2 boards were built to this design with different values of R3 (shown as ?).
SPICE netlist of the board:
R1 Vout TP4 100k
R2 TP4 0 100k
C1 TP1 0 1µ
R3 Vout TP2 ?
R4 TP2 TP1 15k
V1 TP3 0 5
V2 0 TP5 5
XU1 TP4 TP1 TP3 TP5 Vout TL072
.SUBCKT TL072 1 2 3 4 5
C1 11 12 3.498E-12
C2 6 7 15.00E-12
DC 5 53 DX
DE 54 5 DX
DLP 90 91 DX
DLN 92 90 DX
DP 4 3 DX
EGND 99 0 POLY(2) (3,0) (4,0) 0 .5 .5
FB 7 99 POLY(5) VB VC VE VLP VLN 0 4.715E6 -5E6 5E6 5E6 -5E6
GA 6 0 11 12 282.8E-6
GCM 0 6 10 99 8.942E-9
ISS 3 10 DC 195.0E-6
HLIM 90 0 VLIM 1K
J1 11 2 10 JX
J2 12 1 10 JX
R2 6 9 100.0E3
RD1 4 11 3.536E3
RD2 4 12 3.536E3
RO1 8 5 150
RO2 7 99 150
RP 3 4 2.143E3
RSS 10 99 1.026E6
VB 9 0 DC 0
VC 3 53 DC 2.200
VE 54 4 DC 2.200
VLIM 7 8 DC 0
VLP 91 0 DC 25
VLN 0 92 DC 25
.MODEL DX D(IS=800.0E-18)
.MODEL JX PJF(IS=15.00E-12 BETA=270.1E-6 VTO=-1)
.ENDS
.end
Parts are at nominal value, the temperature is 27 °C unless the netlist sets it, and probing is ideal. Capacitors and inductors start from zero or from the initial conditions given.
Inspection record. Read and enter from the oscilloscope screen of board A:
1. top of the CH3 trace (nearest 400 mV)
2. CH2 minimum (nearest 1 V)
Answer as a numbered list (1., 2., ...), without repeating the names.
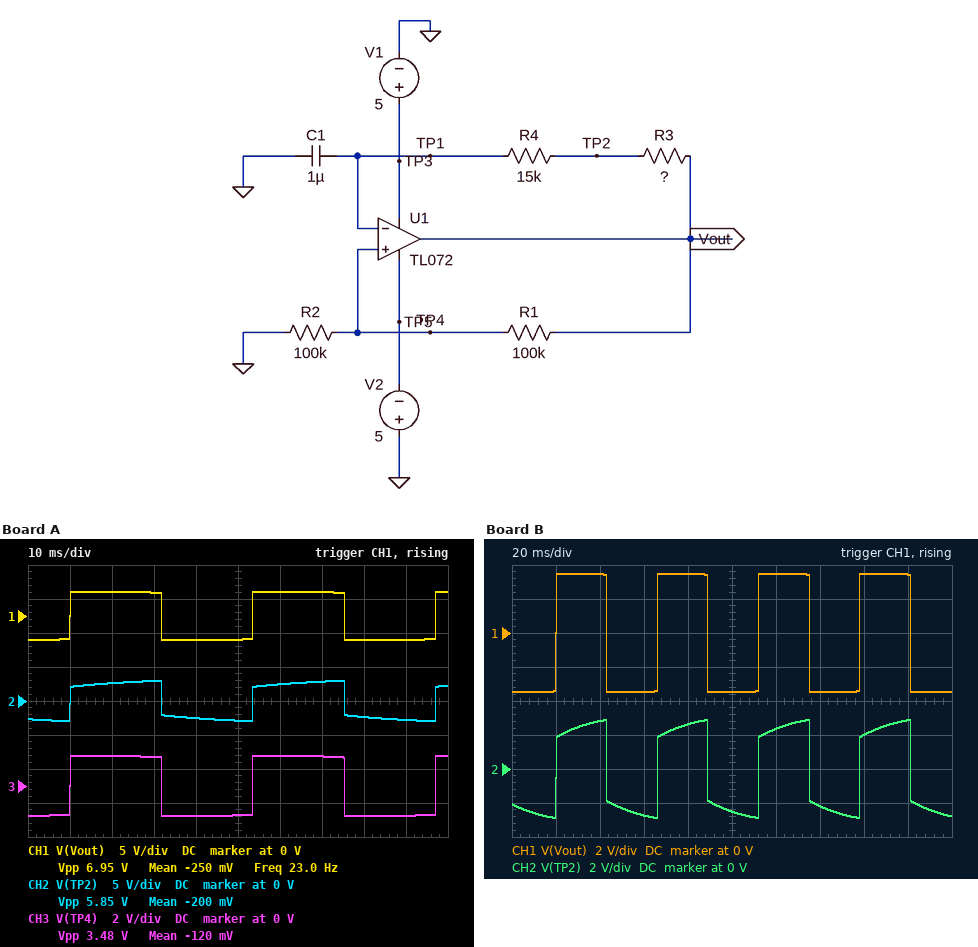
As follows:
1. 1.6 V
2. -3 V
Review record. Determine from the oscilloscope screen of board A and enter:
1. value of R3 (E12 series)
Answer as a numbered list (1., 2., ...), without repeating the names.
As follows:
1. 5.6 kΩ
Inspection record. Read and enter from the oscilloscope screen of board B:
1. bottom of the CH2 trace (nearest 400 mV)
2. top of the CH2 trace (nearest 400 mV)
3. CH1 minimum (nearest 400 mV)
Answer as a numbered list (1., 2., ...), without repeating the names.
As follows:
1. -2.8 V
2. 2.8 V
3. -3.6 V
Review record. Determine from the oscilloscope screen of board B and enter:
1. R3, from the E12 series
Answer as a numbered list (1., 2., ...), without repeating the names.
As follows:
1. 6.8 kΩ
